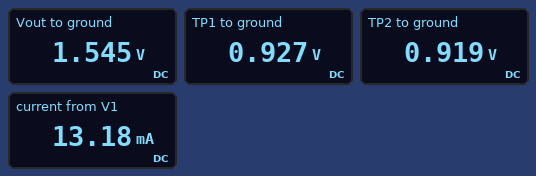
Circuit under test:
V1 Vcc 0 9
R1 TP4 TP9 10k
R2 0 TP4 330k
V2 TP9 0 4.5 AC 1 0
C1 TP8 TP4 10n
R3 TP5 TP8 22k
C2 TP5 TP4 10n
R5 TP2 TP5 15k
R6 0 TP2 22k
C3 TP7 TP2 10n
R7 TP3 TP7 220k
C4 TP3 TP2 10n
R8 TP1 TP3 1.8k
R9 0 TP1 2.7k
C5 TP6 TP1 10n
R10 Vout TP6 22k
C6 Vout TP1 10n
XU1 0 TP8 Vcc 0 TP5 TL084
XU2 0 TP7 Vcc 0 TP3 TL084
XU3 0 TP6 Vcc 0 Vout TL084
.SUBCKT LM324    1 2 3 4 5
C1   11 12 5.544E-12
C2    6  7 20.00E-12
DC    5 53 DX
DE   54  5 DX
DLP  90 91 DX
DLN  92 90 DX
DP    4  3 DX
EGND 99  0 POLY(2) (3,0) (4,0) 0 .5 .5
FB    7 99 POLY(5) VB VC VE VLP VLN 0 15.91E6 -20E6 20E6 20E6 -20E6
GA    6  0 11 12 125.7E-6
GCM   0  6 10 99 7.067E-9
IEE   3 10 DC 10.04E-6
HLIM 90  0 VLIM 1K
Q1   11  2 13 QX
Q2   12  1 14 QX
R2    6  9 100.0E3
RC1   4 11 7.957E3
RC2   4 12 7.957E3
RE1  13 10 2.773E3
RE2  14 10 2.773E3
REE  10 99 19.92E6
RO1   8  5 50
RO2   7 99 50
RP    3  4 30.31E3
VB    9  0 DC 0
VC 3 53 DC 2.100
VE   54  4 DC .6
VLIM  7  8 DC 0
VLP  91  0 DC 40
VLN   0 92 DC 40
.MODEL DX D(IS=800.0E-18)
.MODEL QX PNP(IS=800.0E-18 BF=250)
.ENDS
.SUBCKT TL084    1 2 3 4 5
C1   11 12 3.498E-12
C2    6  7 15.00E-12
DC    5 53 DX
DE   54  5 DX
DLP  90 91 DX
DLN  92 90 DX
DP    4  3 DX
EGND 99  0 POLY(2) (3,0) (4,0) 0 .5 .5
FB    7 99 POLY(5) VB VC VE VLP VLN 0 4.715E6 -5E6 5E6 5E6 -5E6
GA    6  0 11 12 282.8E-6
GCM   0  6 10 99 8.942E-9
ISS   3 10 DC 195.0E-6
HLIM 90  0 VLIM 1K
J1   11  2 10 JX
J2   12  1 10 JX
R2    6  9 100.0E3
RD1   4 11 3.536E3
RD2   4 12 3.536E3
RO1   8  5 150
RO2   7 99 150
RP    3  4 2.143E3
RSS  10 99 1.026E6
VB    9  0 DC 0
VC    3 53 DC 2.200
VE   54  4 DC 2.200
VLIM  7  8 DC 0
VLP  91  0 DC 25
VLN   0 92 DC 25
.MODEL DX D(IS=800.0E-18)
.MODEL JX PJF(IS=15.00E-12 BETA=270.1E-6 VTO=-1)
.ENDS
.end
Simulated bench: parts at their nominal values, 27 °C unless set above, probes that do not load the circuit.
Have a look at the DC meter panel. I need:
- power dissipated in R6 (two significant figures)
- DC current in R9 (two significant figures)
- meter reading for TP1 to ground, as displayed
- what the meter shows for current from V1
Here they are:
38 µW
340 µA
0.927 V
13.18 mA
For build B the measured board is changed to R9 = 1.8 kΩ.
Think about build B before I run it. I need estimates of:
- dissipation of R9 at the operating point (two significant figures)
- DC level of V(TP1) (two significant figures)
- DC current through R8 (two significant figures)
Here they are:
330 µW
770 mV
430 µA
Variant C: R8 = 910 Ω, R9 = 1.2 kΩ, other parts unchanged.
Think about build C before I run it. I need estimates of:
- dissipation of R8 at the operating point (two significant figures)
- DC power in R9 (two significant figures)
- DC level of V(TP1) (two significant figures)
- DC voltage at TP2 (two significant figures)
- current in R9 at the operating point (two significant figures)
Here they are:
490 µW
640 µW
880 mV
920 mV
730 µA
